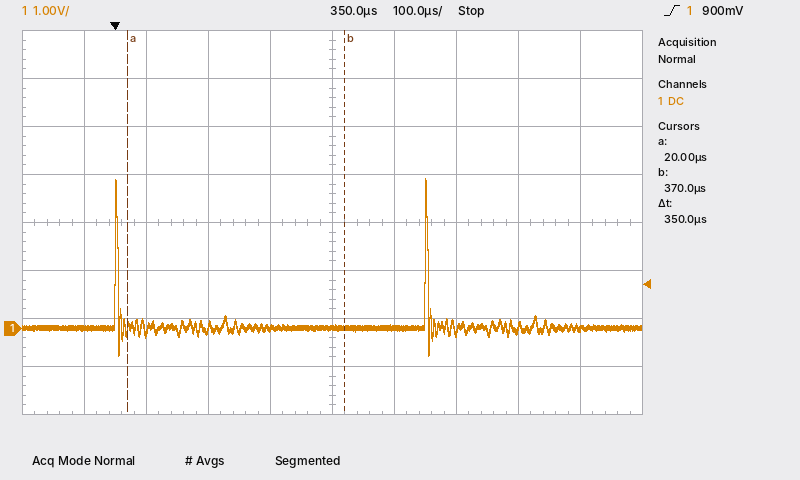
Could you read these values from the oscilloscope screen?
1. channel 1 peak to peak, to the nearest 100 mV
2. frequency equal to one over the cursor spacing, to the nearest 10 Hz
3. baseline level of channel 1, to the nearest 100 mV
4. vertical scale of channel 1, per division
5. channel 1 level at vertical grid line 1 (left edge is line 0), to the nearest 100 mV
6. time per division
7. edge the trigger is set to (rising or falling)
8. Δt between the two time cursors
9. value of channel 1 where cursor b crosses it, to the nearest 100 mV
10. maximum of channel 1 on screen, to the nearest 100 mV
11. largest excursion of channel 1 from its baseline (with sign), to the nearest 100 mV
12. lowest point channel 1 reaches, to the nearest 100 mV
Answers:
3.7 V
2.86 kHz
0.0 V
1 V
0.0 V
100 µs
rising
350 µs
0.0 V
3.1 V
+3.1 V
-600 mV
